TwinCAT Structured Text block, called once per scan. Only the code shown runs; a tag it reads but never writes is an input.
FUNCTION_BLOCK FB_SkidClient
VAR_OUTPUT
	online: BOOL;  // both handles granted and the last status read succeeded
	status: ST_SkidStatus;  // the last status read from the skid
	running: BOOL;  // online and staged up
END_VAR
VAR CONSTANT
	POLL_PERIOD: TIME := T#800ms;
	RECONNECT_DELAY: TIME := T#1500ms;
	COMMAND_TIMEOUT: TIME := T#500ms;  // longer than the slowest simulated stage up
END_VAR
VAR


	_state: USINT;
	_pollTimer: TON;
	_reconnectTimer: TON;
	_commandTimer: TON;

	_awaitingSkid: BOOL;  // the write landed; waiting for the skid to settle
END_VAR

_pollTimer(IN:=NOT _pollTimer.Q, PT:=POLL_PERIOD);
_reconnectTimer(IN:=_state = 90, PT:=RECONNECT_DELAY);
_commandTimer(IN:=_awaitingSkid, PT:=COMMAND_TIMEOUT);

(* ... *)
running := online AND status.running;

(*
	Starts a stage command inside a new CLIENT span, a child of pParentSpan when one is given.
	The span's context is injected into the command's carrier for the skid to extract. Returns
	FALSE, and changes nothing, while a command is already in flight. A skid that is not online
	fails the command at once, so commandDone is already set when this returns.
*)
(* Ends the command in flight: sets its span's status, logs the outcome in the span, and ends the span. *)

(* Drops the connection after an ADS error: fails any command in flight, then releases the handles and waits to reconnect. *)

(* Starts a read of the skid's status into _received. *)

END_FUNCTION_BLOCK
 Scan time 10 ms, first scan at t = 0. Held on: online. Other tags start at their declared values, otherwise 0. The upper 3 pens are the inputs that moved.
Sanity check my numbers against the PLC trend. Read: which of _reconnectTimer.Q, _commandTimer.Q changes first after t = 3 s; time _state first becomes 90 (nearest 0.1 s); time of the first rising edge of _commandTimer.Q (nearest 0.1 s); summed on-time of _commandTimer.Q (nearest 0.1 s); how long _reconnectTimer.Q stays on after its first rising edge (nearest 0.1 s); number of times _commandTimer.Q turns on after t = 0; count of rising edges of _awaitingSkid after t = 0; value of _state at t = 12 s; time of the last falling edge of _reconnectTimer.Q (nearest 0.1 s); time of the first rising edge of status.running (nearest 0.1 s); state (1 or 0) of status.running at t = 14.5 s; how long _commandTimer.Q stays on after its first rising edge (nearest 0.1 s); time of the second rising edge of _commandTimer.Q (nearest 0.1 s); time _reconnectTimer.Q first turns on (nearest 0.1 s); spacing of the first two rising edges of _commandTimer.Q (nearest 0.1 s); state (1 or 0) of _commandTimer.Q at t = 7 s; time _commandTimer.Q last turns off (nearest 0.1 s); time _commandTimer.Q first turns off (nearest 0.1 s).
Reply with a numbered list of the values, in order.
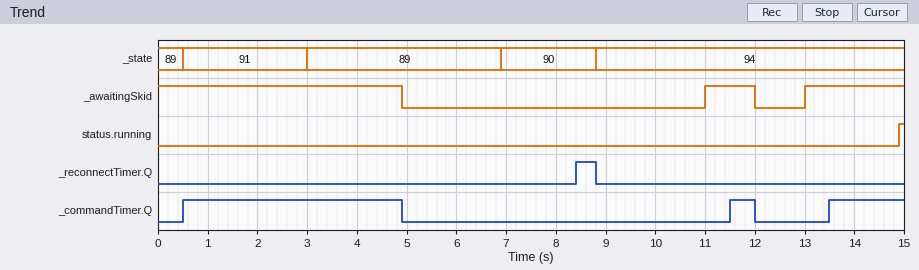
1. _commandTimer.Q
2. 6.9 s
3. 0.5 s
4. 6.4 s
5. 0.4 s
6. 3
7. 2
8. 94
9. 8.8 s
10. 14.9 s
11. 0
12. 4.4 s
13. 11.5 s
14. 8.4 s
15. 11.0 s
16. 0
17. 12.0 s
18. 4.9 s
